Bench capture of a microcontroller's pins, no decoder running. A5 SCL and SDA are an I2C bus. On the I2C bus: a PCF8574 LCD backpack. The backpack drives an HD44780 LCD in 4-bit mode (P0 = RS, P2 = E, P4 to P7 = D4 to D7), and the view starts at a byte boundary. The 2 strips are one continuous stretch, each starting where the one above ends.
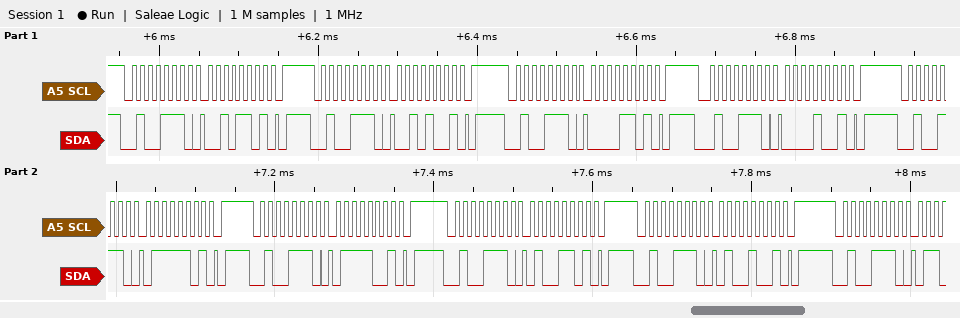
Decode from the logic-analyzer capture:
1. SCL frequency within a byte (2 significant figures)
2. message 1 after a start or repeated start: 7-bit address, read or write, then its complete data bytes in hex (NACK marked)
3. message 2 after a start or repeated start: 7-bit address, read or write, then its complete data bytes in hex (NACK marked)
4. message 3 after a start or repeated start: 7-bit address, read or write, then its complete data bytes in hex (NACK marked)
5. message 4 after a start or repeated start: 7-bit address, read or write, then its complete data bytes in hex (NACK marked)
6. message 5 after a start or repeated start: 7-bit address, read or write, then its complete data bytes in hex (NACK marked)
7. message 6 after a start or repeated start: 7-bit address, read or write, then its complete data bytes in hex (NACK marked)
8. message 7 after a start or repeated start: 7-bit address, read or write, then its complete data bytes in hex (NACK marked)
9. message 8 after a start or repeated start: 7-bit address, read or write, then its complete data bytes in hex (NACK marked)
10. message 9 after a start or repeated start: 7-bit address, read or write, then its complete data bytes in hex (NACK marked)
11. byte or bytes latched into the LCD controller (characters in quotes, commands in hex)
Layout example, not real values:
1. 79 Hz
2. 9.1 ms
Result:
1. 100 kHz
2. 0x27 write: 2D
3. 0x27 write: 29
4. 0x27 write: 0D
5. 0x27 write: 09
6. 0x27 write: 7D
7. 0x27 write: 79
8. 0x27 write: 4D
9. 0x27 write: 49
10. 0x27 write
11. ' ' 't'
